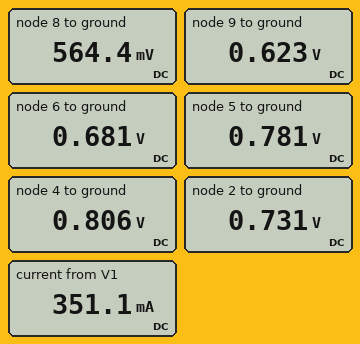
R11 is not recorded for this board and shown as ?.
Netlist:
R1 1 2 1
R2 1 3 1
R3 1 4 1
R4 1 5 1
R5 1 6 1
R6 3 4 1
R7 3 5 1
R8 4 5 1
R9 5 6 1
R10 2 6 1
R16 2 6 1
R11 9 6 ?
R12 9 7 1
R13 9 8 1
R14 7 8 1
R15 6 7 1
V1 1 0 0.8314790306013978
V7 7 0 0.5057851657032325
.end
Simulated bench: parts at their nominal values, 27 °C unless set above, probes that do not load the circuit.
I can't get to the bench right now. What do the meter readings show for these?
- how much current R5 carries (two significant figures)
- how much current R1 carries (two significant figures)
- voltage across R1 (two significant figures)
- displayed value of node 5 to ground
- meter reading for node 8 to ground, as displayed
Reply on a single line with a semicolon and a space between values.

150 mA; 100 mA; 100 mV; 0.781 V; 564.4 mV
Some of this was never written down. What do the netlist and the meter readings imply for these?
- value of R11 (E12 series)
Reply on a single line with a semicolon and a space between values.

0.33 Ω
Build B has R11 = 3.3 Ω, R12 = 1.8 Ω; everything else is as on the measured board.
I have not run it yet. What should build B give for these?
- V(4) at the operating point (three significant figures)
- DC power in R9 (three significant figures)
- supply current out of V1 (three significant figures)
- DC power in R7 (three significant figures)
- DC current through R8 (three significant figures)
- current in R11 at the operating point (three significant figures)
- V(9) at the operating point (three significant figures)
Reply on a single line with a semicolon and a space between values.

813 mV; 5.65 mW; 263 mA; 353 µW; 18.8 mA; 50.1 mA; 553 mV
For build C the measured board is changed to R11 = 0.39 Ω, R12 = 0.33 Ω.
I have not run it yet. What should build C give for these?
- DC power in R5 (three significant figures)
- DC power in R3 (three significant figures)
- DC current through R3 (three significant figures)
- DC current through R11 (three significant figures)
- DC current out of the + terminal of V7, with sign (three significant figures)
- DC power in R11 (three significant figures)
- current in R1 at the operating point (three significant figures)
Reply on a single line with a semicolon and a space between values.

28.2 mW; 784 µW; 28.0 mA; 234 mA; -392 mA; 21.4 mW; 112 mA
